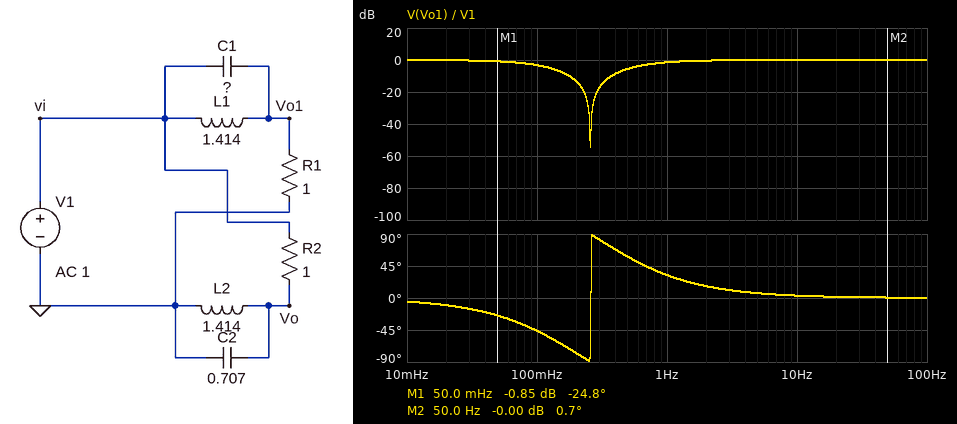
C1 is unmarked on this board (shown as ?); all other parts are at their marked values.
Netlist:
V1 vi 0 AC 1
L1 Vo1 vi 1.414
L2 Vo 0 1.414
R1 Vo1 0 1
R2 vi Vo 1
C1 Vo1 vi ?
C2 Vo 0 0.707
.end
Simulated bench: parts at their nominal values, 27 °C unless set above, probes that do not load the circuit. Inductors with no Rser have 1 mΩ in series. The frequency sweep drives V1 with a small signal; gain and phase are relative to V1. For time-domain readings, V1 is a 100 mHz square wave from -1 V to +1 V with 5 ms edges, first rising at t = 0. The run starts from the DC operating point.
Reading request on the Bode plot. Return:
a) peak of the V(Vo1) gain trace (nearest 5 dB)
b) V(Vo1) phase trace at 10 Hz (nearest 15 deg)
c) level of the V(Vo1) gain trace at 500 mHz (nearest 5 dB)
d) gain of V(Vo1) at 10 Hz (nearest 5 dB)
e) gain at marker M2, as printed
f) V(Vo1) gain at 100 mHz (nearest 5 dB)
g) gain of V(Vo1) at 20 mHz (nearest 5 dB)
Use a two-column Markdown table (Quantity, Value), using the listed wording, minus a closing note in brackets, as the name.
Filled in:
| Quantity | Value |
|---|---|
| peak of the V(Vo1) gain trace | 0 dB |
| V(Vo1) phase trace at 10 Hz | 0 deg |
| level of the V(Vo1) gain trace at 500 mHz | -5 dB |
| gain of V(Vo1) at 10 Hz | 0 dB |
| gain at marker M2, as printed | -0.00 dB |
| V(Vo1) gain at 100 mHz | -5 dB |
| gain of V(Vo1) at 20 mHz | 0 dB |
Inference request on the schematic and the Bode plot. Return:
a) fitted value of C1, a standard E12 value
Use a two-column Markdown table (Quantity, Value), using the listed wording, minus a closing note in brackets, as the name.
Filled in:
| Quantity | Value |
|---|---|
| fitted value of C1, a standard E12 value | 270 mF |
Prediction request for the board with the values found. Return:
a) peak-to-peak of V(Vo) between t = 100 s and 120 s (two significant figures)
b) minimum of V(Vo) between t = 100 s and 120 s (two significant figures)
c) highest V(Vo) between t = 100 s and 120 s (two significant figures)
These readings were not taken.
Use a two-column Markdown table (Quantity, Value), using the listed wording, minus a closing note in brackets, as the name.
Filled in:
| Quantity | Value |
|---|---|
| peak-to-peak of V(Vo) between t = 100 s and 120 s | 2.7 V |
| minimum of V(Vo) between t = 100 s and 120 s | -1.3 V |
| highest V(Vo) between t = 100 s and 120 s | 1.3 V |
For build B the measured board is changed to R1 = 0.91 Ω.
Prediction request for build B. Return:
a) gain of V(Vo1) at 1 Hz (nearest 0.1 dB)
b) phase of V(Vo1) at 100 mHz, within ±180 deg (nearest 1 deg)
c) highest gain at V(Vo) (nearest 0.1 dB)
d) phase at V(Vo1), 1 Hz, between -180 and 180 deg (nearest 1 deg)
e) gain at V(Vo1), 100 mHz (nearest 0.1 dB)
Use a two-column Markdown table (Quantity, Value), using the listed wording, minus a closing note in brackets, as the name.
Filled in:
| Quantity | Value |
|---|---|
| gain of V(Vo1) at 1 Hz | -1.7 dB |
| phase of V(Vo1) at 100 mHz, within ±180 deg | -49 deg |
| highest gain at V(Vo) | 0 dB |
| phase at V(Vo1), 1 Hz, between -180 and 180 deg | 35 deg |
| gain at V(Vo1), 100 mHz | -3.7 dB |
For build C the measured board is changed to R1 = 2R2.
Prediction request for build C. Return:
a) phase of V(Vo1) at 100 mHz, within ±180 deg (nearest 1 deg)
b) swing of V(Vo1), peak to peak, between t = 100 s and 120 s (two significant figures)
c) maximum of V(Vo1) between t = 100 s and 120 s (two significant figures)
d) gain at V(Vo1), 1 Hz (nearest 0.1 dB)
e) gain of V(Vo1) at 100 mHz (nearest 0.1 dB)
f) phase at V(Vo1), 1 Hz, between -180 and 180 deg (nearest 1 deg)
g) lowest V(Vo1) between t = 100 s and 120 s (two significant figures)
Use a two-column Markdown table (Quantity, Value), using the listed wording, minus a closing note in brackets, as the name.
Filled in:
| Quantity | Value |
|---|---|
| phase of V(Vo1) at 100 mHz, within ±180 deg | -25 deg |
| swing of V(Vo1), peak to peak, between t = 100 s and 120 s | 2.3 V |
| maximum of V(Vo1) between t = 100 s and 120 s | 1.2 V |
| gain at V(Vo1), 1 Hz | -0.3 dB |
| gain of V(Vo1) at 100 mHz | -0.9 dB |
| phase at V(Vo1), 1 Hz, between -180 and 180 deg | 16 deg |
| lowest V(Vo1) between t = 100 s and 120 s | -1.2 V |
